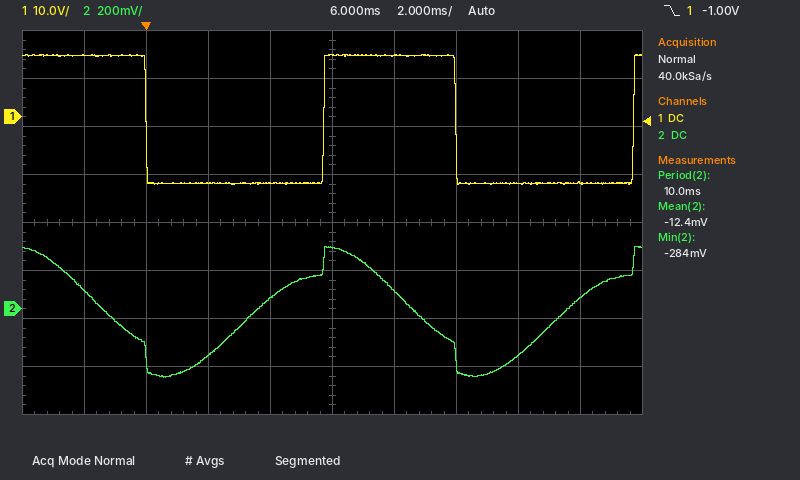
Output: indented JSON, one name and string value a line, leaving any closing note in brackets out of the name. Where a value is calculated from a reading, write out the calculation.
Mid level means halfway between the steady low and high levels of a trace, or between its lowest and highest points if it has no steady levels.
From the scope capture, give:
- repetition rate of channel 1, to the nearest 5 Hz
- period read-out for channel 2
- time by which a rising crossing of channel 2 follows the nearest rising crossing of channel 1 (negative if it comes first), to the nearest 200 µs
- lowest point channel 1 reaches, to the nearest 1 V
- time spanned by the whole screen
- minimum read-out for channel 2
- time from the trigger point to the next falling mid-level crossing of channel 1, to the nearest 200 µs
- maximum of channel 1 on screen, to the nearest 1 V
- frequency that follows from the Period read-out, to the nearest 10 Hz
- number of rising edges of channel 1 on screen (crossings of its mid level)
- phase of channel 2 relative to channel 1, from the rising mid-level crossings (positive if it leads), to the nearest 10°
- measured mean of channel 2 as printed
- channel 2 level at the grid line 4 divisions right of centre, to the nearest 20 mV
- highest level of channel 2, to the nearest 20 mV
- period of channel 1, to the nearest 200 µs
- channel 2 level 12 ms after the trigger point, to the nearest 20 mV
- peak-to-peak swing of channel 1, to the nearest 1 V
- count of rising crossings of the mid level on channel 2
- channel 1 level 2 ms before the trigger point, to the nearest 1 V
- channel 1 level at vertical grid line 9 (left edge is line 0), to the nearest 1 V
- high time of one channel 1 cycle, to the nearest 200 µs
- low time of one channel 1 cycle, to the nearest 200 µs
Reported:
{
  "repetition rate of channel 1, to the nearest 5 Hz": "1 / 10.0 ms ≈ 100 Hz",
  "period read-out for channel 2": "10.0 ms",
  "time by which a rising crossing of channel 2 follows the nearest rising crossing of channel 1 (negative if it comes first), to the nearest 200 µs": "-2.2 ms",
  "lowest point channel 1 reaches, to the nearest 1 V": "-14 V",
  "time spanned by the whole screen": "20 ms",
  "minimum read-out for channel 2": "-284 mV",
  "time from the trigger point to the next falling mid-level crossing of channel 1, to the nearest 200 µs": "10.0 ms",
  "maximum of channel 1 on screen, to the nearest 1 V": "13 V",
  "frequency that follows from the Period read-out, to the nearest 10 Hz": "1 / 10.0 ms ≈ 100 Hz",
  "number of rising edges of channel 1 on screen": "2",
  "phase of channel 2 relative to channel 1, from the rising mid-level crossings (positive if it leads), to the nearest 10°": "−360° × (-2.2 ms) / 10.0 ms ≈ +79.2°, so +80° to the nearest 10°",
  "measured mean of channel 2 as printed": "-12.4 mV",
  "channel 2 level at the grid line 4 divisions right of centre, to the nearest 20 mV": "40 mV",
  "highest level of channel 2, to the nearest 20 mV": "260 mV",
  "period of channel 1, to the nearest 200 µs": "10.0 ms",
  "channel 2 level 12 ms after the trigger point, to the nearest 20 mV": "-200 mV",
  "peak-to-peak swing of channel 1, to the nearest 1 V": "13 V − (-14 V) = 27 V",
  "count of rising crossings of the mid level on channel 2": "2",
  "channel 1 level 2 ms before the trigger point, to the nearest 1 V": "13 V",
  "channel 1 level at vertical grid line 9 (left edge is line 0), to the nearest 1 V": "-14 V",
  "high time of one channel 1 cycle, to the nearest 200 µs": "4.2 ms",
  "low time of one channel 1 cycle, to the nearest 200 µs": "5.8 ms"
}
